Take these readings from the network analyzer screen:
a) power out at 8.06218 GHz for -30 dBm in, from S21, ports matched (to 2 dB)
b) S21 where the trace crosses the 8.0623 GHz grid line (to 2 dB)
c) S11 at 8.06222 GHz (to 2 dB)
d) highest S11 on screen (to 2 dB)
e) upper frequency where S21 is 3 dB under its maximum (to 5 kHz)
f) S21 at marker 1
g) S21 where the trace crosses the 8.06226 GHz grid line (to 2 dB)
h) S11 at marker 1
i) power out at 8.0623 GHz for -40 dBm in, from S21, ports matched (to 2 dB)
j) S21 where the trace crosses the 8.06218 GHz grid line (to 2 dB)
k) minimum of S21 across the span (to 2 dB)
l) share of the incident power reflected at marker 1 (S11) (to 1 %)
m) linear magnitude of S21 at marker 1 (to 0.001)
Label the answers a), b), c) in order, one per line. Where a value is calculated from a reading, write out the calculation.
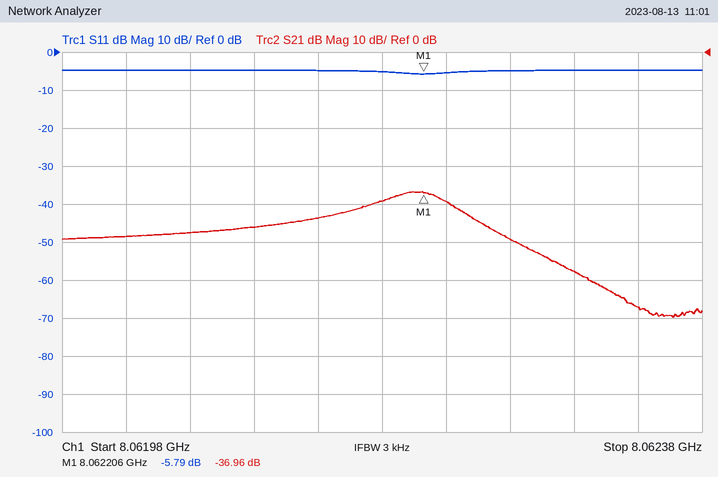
a) -30 dBm + (-40 dB) = -70 dBm
b) -58 dB
c) -6 dB
d) -4 dB
e) 8.062220 GHz
f) -36.96 dB
g) -50 dB
h) -5.79 dB
i) -40 dBm + (-58 dB) = -98 dBm
j) -40 dB
k) -70 dB
l) 10^(-5.79/10) ≈ 26 %
m) 10^(-36.96/20) ≈ 0.014
